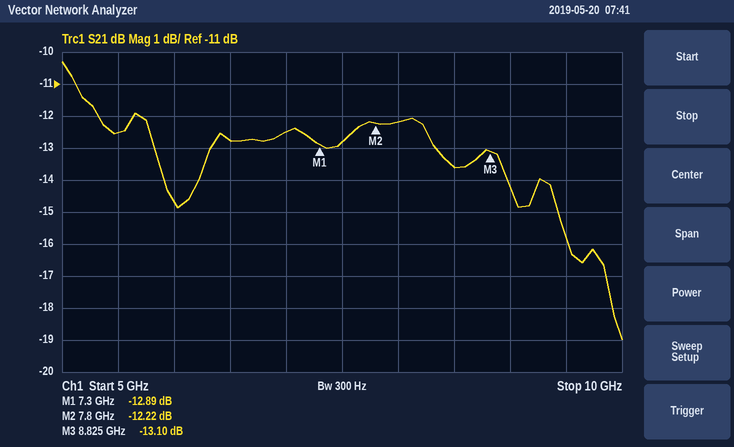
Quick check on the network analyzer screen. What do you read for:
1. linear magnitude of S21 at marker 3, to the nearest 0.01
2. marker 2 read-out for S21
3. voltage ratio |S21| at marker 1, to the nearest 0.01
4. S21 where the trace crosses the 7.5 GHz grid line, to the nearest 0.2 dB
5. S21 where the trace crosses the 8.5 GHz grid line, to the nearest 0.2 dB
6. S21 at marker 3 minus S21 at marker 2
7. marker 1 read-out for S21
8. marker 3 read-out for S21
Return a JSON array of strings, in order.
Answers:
["0.22", "-12.22 dB", "0.23", "-12.8 dB", "-13.6 dB", "-0.88 dB", "-12.89 dB", "-13.10 dB"]
